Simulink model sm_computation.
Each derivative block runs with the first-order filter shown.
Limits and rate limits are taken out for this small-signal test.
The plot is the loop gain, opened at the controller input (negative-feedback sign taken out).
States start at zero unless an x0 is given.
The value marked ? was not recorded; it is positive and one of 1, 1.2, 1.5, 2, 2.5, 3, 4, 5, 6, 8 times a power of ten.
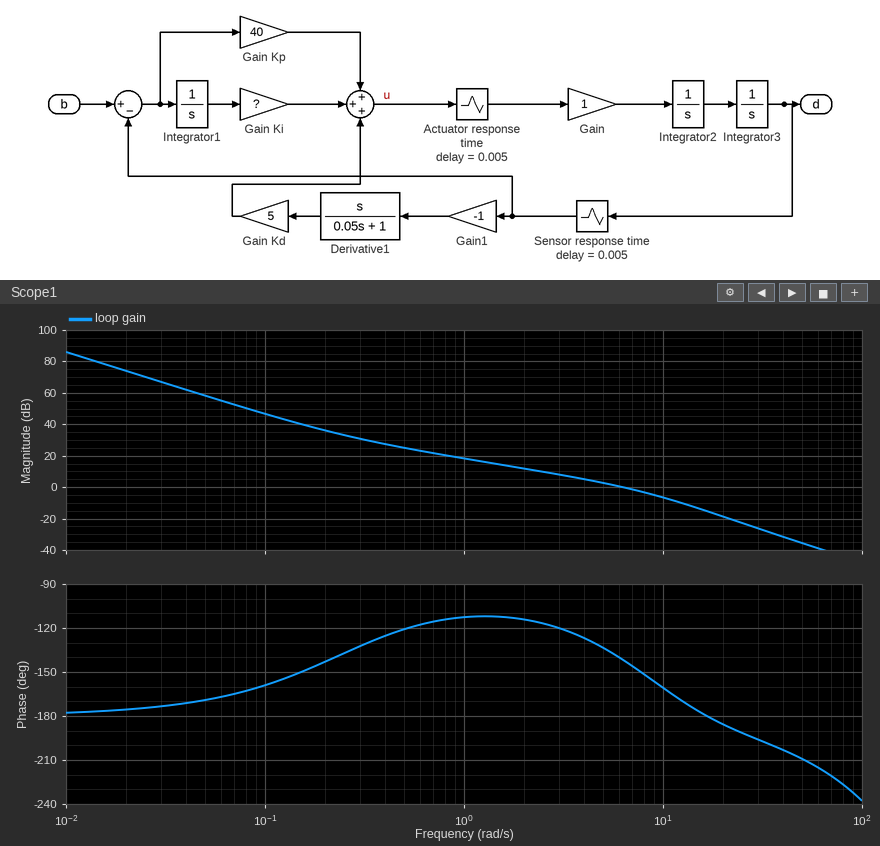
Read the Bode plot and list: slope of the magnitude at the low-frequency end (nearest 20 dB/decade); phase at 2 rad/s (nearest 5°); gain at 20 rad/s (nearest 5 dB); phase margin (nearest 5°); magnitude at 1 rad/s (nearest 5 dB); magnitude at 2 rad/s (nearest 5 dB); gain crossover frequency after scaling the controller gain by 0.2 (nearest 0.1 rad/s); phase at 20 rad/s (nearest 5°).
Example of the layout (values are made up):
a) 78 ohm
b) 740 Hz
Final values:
a) -40 dB/decade
b) -115°
c) -20 dB
d) 40°
e) 20 dB
f) 10 dB
g) 1.6 rad/s
h) -185°
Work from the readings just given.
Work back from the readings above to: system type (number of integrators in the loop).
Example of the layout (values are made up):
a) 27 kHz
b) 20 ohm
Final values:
a) 2
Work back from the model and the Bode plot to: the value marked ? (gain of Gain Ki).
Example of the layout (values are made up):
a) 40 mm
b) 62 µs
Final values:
a) 10
